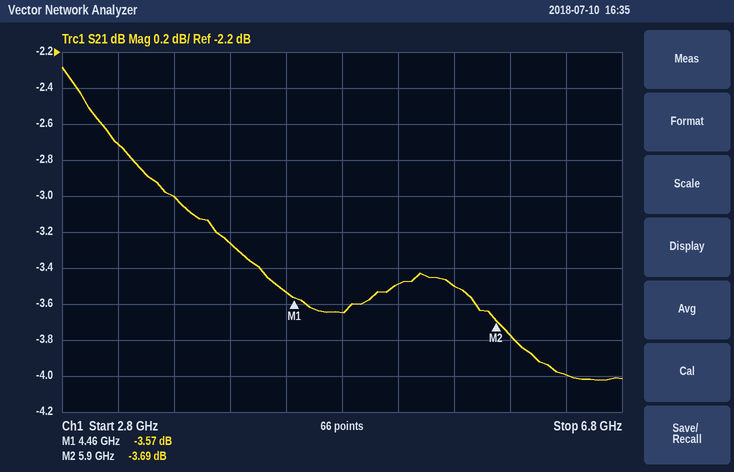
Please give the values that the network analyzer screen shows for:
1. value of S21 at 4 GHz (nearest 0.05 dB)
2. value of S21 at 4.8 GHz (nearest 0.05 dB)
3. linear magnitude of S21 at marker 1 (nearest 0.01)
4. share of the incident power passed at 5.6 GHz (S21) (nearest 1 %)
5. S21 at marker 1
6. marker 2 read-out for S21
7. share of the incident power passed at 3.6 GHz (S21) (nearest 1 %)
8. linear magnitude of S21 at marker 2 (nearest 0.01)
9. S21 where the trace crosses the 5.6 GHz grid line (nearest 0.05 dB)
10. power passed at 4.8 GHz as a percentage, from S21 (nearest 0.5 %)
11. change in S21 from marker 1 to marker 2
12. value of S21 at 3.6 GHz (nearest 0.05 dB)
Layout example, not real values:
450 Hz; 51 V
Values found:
-3.25 dB; -3.65 dB; 0.66; 45 %; -3.57 dB; -3.69 dB; 50 %; 0.65; -3.50 dB; 43.0 %; -0.12 dB; -3.00 dB
